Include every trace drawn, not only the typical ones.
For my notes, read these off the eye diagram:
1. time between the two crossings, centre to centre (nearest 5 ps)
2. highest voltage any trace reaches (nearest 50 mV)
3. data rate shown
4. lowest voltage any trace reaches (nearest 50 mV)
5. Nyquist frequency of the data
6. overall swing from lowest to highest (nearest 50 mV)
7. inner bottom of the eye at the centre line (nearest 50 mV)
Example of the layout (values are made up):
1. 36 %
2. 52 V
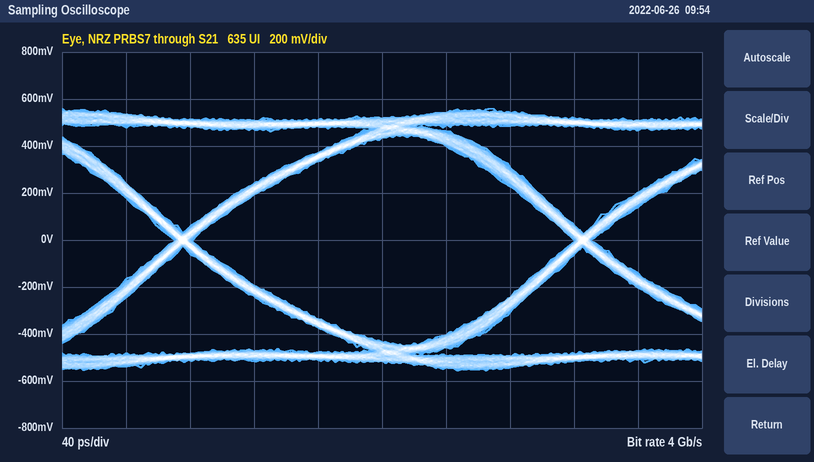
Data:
1. 250 ps
2. 550 mV
3. 4 Gb/s
4. -550 mV
5. 2 GHz
6. 1.10 V
7. -450 mV
